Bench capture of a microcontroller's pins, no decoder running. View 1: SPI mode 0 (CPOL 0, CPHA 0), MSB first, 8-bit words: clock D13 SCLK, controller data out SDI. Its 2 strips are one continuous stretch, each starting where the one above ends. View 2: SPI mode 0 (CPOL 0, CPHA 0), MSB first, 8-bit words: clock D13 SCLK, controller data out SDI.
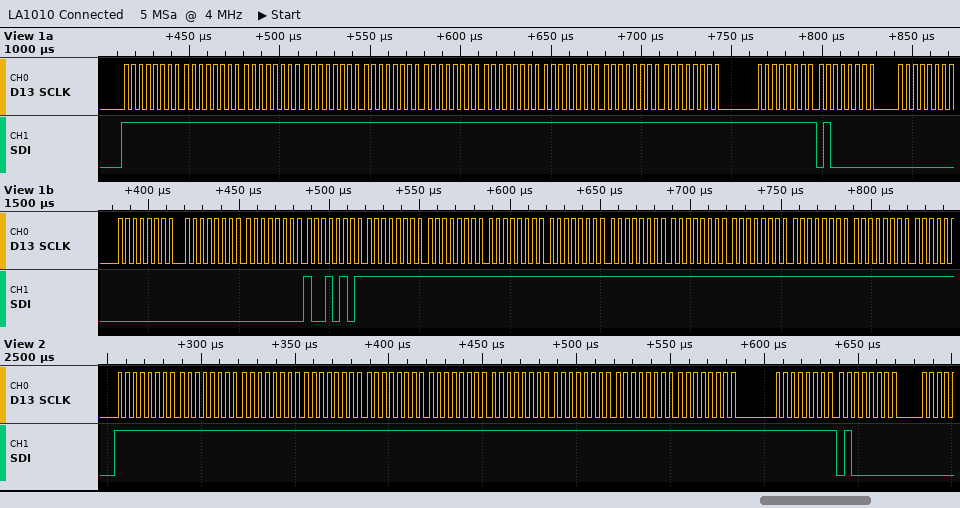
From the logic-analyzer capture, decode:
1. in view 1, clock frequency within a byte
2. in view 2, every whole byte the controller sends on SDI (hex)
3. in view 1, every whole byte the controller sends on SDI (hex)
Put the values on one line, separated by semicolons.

250 kHz; 0xFF 0xFF 0xFF 0xFF 0xFF 0xFF 0xFF 0xFF 0xFF 0xFF 0xFF 0x40; FF FF FF FF FF FF FF FF FF FF FF 40 00 00 00 00 95 FF FF FF FF FF FF FF FF FF
